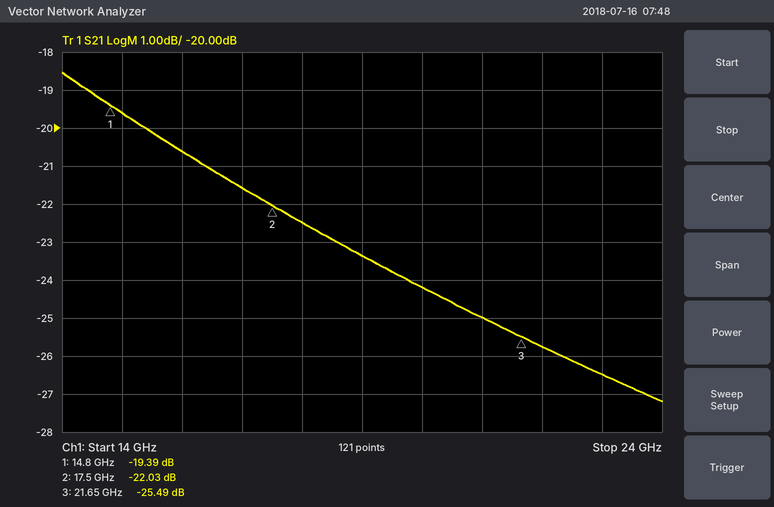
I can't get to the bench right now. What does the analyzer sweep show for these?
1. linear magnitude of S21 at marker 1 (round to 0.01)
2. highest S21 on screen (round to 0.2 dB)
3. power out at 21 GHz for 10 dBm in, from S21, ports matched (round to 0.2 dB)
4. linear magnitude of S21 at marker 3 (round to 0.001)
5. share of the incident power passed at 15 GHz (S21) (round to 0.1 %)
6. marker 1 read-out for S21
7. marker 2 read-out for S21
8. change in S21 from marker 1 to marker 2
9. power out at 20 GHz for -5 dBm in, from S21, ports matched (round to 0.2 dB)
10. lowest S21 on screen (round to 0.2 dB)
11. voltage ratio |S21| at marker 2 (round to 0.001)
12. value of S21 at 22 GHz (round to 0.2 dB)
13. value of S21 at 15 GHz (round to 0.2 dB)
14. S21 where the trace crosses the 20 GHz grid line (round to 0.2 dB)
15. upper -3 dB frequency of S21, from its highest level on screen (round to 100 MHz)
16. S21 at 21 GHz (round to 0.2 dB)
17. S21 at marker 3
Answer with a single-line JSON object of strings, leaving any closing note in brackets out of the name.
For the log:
{"linear magnitude of S21 at marker 1": "0.11", "highest S21 on screen": "-18.6 dB", "power out at 21 GHz for 10 dBm in, from S21, ports matched": "-15.0 dBm", "linear magnitude of S21 at marker 3": "0.053", "share of the incident power passed at 15 GHz (S21)": "1.1 %", "marker 1 read-out for S21": "-19.39 dB", "marker 2 read-out for S21": "-22.03 dB", "change in S21 from marker 1 to marker 2": "-2.64 dB", "power out at 20 GHz for -5 dBm in, from S21, ports matched": "-29.2 dBm", "lowest S21 on screen": "-27.2 dB", "voltage ratio |S21| at marker 2": "0.079", "value of S21 at 22 GHz": "-25.8 dB", "value of S21 at 15 GHz": "-19.6 dB", "S21 where the trace crosses the 20 GHz grid line": "-24.2 dB", "upper -3 dB frequency of S21, from its highest level on screen": "17.0 GHz", "S21 at 21 GHz": "-25.0 dB", "S21 at marker 3": "-25.49 dB"}
